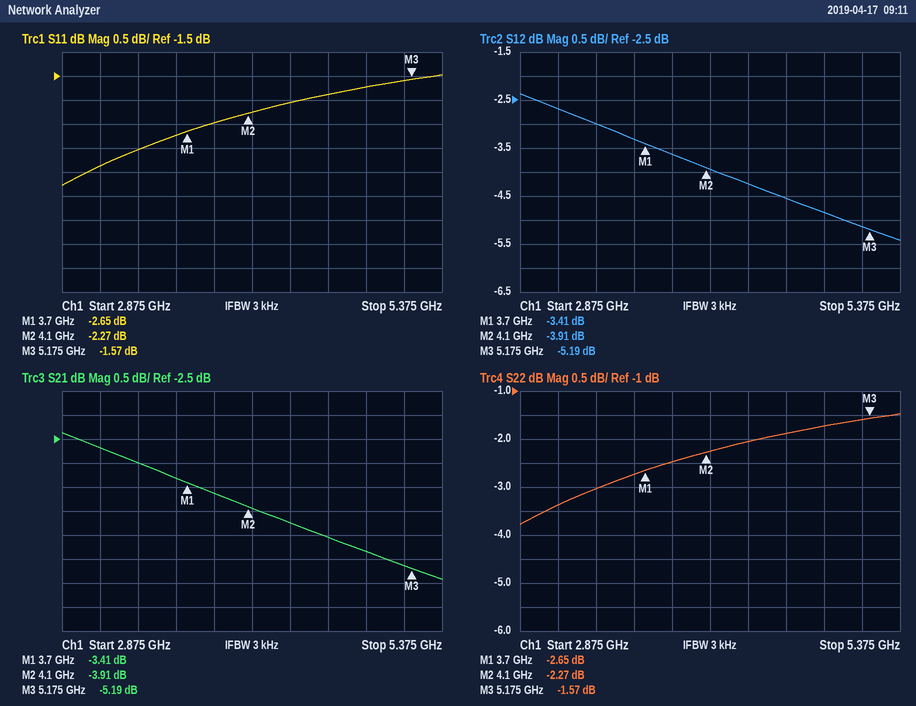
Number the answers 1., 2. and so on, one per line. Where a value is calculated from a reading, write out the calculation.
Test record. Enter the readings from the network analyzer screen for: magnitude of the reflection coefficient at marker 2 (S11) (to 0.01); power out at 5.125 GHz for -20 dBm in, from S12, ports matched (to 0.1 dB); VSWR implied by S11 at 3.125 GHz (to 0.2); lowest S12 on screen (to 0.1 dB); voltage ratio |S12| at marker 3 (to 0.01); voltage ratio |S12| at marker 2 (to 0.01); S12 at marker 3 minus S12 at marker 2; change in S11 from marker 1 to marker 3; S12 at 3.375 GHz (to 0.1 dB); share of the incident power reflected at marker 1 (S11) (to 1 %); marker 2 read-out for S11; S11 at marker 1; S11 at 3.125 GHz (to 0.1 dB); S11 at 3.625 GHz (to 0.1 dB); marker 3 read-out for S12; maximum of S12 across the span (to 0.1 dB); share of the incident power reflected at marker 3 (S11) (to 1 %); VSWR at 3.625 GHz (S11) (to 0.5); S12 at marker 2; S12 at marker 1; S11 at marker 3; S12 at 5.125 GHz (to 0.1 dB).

1. 10^(-2.27/20) ≈ 0.77
2. -20 dBm + (-5.1 dB) = -25.1 dBm
3. |Γ| = 10^(-3.4/20) = 0.6761; VSWR = (1 + 0.6761)/(1 − 0.6761) ≈ 5.2
4. -5.4 dB
5. 10^(-5.19/20) ≈ 0.55
6. 10^(-3.91/20) ≈ 0.64
7. -5.19 − (-3.91) = -1.28 dB
8. -1.57 − (-2.65) = 1.08 dB
9. -3.0 dB
10. 10^(-2.65/10) ≈ 54 %
11. -2.27 dB
12. -2.65 dB
13. -3.4 dB
14. -2.7 dB
15. -5.19 dB
16. -2.4 dB
17. 10^(-1.57/10) ≈ 70 %
18. |Γ| = 10^(-2.7/20) = 0.7328; VSWR = (1 + 0.7328)/(1 − 0.7328) ≈ 6.5
19. -3.91 dB
20. -3.41 dB
21. -1.57 dB
22. -5.1 dB
